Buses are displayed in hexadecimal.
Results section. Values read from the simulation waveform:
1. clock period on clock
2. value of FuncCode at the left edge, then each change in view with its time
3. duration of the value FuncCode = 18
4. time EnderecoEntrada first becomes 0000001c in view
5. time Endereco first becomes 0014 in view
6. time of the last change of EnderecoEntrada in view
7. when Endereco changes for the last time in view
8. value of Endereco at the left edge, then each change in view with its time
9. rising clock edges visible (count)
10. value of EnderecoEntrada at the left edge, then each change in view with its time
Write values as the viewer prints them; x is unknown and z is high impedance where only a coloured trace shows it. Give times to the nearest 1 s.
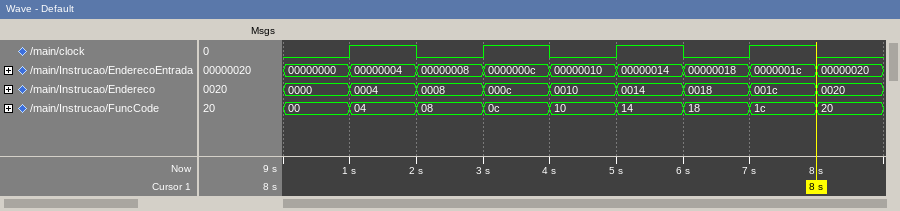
2 s
00, 04 at 1 s, 08 at 2 s, 0c at 3 s, 10 at 4 s, 14 at 5 s, 18 at 6 s, 1c at 7 s, 20 at 8 s
1 s
7 s
5 s
8 s
8 s
0000, 0004 at 1 s, 0008 at 2 s, 000c at 3 s, 0010 at 4 s, 0014 at 5 s, 0018 at 6 s, 001c at 7 s, 0020 at 8 s
4
00000000, 00000004 at 1 s, 00000008 at 2 s, 0000000c at 3 s, 00000010 at 4 s, 00000014 at 5 s, 00000018 at 6 s, 0000001c at 7 s, 00000020 at 8 s
